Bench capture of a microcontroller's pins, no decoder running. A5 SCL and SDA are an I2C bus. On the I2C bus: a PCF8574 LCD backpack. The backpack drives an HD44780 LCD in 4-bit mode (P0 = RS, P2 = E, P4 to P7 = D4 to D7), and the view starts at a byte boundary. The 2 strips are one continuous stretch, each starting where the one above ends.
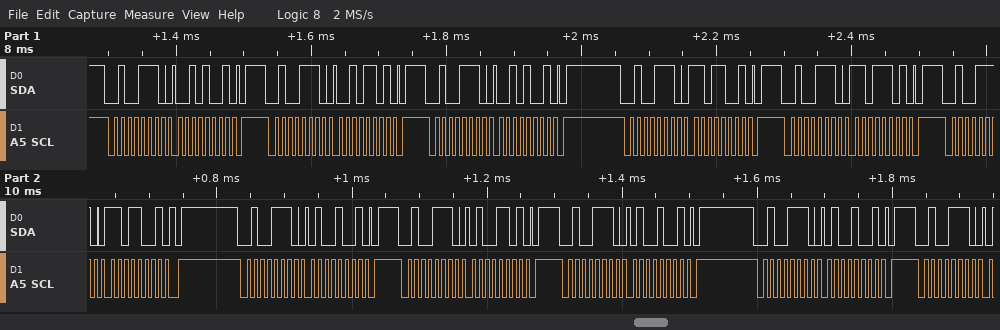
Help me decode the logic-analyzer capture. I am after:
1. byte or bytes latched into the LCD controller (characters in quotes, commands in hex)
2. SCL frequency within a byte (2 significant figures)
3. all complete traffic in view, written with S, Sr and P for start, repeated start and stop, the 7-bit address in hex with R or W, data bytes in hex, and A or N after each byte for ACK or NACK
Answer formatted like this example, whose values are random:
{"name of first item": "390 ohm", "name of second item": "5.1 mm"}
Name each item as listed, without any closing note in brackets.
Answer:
{"byte or bytes latched into the LCD controller": "'-'", "SCL frequency within a byte": "100 kHz", "all complete traffic in view, written with S, Sr and P for start, repeated start and stop, the 7-bit address in hex with R or W, data bytes in hex, and A or N after each byte for ACK or NACK": "S 27W A 29 A P S 27W A 2D A P S 27W A 29 A P S 27W A D9 A P S 27W A DD A P S 27W A D9 A P S 27W A 49 A P S 27W A 4D A P S 27W A 49 A P S 27W A 49 A P S 27W A"}
